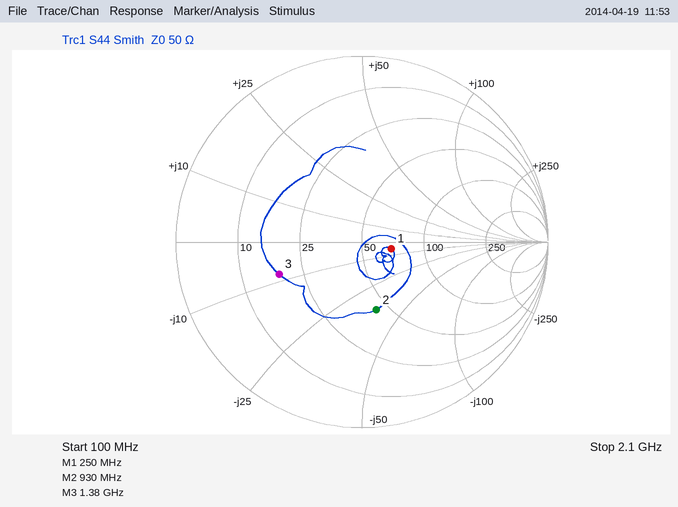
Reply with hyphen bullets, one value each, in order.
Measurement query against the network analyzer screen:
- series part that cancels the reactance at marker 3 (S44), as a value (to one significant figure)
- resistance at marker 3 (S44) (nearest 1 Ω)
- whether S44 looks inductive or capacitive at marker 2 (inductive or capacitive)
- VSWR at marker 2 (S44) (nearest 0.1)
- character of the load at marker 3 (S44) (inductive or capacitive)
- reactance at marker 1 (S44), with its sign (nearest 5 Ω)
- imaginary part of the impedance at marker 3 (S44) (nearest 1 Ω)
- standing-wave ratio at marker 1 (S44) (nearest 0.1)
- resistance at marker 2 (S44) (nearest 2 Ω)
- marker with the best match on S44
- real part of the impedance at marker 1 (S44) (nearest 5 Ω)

- 900 pH
- 18 Ω
- capacitive
- 2.2
- capacitive
- -5 Ω
- -8 Ω
- 1.4
- 44 Ω
- marker 1
- 70 Ω
